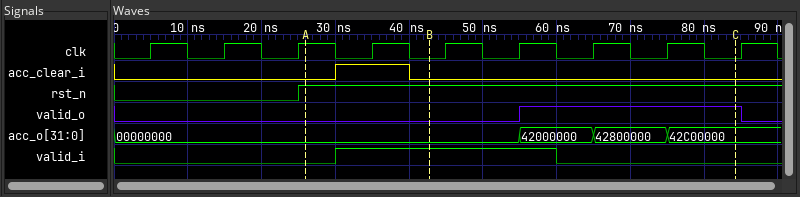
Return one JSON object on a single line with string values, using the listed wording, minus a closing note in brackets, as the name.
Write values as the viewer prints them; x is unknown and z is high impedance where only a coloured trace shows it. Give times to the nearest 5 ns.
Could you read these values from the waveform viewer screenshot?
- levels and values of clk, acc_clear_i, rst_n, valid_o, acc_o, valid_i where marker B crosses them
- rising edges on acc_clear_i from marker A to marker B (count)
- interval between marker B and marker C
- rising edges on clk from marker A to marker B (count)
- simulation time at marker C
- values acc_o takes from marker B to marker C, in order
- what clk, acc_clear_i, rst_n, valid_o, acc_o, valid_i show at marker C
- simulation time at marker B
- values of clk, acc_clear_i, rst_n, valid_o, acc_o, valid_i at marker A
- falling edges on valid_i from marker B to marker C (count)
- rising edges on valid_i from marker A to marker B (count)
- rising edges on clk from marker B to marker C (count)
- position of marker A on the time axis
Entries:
{"levels and values of clk, acc_clear_i, rst_n, valid_o, acc_o, valid_i where marker B crosses them": "clk=0, acc_clear_i=0, rst_n=1, valid_o=0, acc_o=00000000, valid_i=1", "rising edges on acc_clear_i from marker A to marker B": "1", "interval between marker B and marker C": "40 ns", "rising edges on clk from marker A to marker B": "1", "simulation time at marker C": "85 ns", "values acc_o takes from marker B to marker C, in order": "00000000, 42000000, 42800000, 42C00000", "what clk, acc_clear_i, rst_n, valid_o, acc_o, valid_i show at marker C": "clk=0, acc_clear_i=0, rst_n=1, valid_o=1, acc_o=42C00000, valid_i=0", "simulation time at marker B": "45 ns", "values of clk, acc_clear_i, rst_n, valid_o, acc_o, valid_i at marker A": "clk=1, acc_clear_i=0, rst_n=1, valid_o=0, acc_o=00000000, valid_i=0", "falling edges on valid_i from marker B to marker C": "1", "rising edges on valid_i from marker A to marker B": "1", "rising edges on clk from marker B to marker C": "4", "position of marker A on the time axis": "25 ns"}
